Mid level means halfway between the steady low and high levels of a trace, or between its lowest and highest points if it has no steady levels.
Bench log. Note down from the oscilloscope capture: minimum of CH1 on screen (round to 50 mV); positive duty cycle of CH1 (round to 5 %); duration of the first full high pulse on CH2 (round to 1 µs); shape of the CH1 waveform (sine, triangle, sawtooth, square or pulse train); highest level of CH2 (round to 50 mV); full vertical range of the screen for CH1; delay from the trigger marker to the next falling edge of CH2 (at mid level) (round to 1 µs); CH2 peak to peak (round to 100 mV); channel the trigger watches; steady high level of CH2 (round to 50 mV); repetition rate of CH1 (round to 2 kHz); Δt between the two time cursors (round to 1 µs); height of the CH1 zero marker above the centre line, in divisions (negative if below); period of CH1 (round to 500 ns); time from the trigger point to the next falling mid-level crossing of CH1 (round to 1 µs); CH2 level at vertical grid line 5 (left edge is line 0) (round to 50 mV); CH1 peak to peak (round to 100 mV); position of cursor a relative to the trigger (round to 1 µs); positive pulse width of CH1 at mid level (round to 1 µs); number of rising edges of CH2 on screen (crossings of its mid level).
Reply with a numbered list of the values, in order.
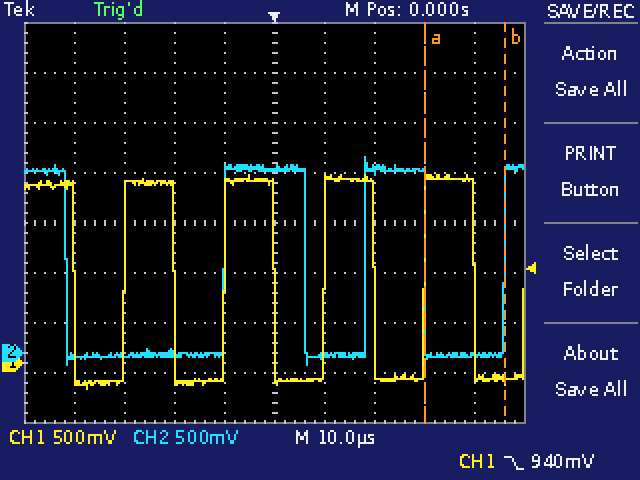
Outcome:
1. -250 mV
2. 50 %
3. 16 µs
4. square
5. 1.95 V
6. 4 V
7. 6 µs
8. 2.10 V
9. CH1
10. 1.85 V
11. 50 kHz
12. 16 µs
13. -2.8 div
14. 20.0 µs
15. 20 µs
16. 1.85 V
17. 2.10 V
18. +30 µs
19. 10 µs
20. 3
